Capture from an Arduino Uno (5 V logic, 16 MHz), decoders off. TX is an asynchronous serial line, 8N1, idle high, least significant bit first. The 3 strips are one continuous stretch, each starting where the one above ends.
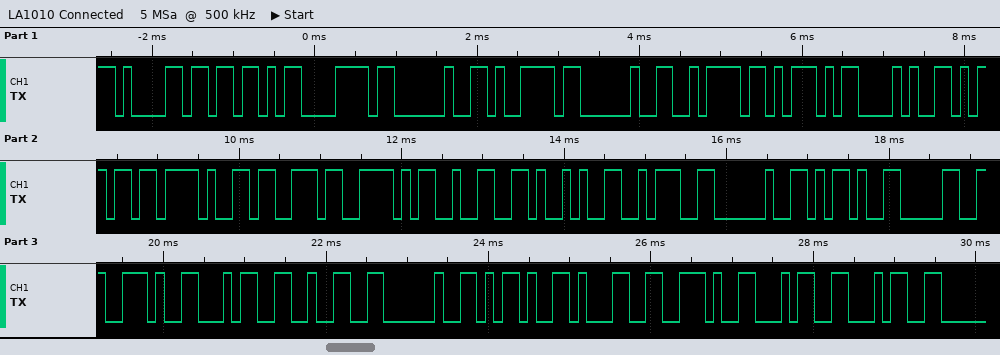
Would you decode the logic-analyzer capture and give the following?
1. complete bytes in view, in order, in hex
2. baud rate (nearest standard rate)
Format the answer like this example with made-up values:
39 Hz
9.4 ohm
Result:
61 5B 78 20 79 20 7A 5D 28 6D 2F 73 5E 32 29 3A 20 2D 30 2E 34 32 20 2D 31 2E 34 34
9600 baud
